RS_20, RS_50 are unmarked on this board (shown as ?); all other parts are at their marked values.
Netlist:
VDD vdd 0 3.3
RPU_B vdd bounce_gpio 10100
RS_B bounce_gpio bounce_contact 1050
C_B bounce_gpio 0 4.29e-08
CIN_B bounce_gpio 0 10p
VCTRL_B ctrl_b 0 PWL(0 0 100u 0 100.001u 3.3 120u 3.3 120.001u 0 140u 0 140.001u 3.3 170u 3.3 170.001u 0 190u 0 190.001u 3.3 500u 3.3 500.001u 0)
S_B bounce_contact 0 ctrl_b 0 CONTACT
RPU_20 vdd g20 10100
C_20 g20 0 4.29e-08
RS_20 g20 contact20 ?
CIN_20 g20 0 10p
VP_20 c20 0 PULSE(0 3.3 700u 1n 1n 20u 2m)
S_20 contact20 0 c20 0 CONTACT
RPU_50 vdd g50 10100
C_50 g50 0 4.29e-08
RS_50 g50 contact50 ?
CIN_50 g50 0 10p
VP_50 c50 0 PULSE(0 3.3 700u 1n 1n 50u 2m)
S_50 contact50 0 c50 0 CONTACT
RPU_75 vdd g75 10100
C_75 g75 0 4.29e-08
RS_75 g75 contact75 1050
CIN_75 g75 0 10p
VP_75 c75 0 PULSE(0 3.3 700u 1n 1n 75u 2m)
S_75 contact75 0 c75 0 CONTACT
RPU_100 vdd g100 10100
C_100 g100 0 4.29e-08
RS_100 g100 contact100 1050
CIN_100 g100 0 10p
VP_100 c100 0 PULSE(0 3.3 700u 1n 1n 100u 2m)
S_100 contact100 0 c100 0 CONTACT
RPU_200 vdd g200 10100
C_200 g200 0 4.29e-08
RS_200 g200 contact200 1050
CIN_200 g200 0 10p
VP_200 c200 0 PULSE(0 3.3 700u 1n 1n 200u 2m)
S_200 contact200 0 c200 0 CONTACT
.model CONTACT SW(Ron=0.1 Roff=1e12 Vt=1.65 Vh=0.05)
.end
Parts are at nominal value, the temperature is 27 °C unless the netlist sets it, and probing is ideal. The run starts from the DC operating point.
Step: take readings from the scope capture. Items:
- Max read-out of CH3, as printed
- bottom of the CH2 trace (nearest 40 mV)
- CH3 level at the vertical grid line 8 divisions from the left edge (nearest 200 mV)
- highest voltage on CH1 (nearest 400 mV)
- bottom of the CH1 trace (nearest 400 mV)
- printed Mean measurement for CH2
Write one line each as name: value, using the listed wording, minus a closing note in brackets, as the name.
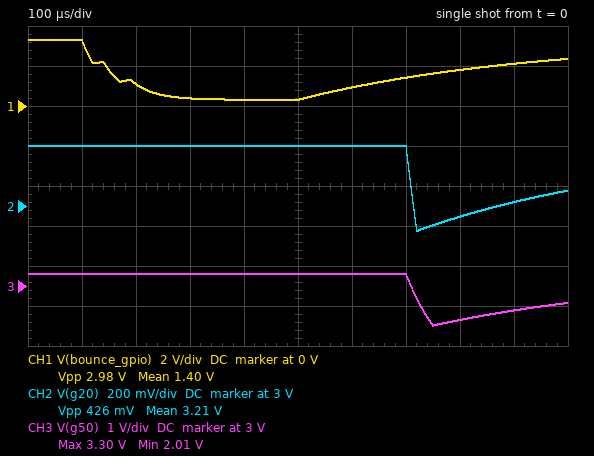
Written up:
Max read-out of CH3, as printed: 3.30 V
bottom of the CH2 trace: 2.88 V
CH3 level at the vertical grid line 8 divisions from the left edge: 2.2 V
highest voltage on CH1: 3.2 V
bottom of the CH1 trace: 400 mV
printed Mean measurement for CH2: 3.21 V
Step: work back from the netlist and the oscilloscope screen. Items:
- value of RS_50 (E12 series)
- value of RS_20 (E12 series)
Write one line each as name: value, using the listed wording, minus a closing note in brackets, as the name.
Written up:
value of RS_50: 2.2 kΩ
value of RS_20: 3.3 kΩ
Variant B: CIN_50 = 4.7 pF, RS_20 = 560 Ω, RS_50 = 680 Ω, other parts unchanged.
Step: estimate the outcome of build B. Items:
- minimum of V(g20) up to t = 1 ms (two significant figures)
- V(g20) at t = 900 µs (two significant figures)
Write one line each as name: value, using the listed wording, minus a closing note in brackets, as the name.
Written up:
minimum of V(g20) up to t = 1 ms: 1.5 V
V(g20) at t = 900 µs: 2.1 V
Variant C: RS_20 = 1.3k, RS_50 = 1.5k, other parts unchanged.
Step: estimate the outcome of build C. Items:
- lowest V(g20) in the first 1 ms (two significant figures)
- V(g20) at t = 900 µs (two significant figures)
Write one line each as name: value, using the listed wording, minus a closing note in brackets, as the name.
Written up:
lowest V(g20) in the first 1 ms: 2.3 V
V(g20) at t = 900 µs: 2.7 V
